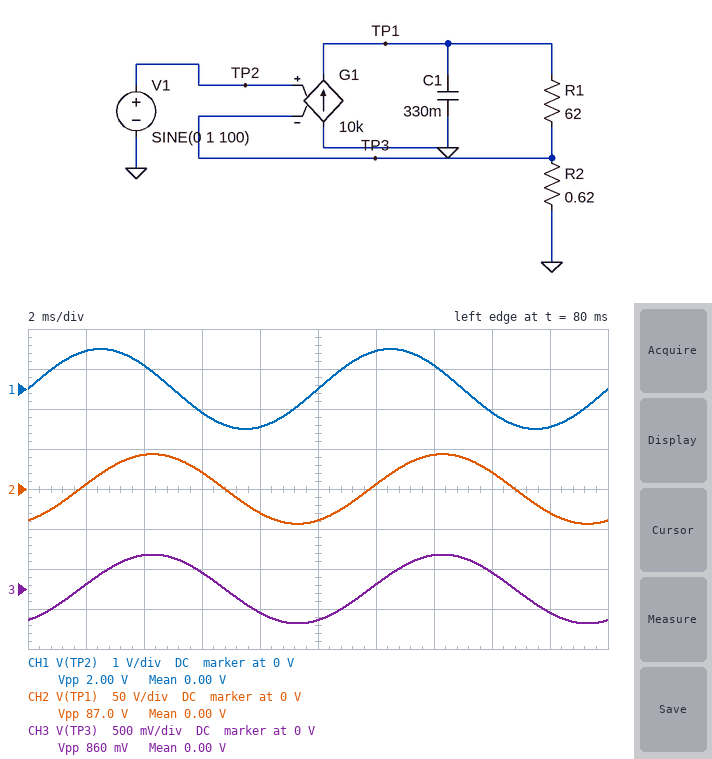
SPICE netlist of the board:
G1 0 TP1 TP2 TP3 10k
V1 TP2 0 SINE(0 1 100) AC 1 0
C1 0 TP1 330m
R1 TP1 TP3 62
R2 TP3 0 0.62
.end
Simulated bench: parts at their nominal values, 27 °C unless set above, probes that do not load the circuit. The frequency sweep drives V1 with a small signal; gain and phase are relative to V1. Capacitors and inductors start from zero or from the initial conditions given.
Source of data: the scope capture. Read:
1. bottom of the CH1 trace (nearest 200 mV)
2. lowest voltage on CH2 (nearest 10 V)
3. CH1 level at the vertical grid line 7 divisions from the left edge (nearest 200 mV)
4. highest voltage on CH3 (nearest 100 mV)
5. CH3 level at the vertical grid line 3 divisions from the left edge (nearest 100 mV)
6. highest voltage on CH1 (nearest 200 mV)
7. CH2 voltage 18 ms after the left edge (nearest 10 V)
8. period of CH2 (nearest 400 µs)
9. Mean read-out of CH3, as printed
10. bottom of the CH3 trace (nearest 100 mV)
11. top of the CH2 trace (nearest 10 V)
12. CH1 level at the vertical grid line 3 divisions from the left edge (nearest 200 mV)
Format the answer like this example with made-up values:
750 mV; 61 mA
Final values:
-1.0 V; -40 V; 600 mV; 400 mV; 200 mV; 1.0 V; -30 V; 10.0 ms; 0.00 V; -400 mV; 40 V; -600 mV
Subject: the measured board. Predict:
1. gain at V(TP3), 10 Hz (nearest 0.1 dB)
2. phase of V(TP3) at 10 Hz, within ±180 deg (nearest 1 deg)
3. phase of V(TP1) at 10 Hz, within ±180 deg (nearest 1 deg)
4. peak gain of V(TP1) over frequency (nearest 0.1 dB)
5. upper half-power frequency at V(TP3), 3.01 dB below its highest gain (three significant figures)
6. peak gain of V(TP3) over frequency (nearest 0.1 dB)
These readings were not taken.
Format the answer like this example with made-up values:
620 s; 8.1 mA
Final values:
-0.2 dB; -12 deg; -12 deg; 40.1 dB; 47.8 Hz; 0 dB
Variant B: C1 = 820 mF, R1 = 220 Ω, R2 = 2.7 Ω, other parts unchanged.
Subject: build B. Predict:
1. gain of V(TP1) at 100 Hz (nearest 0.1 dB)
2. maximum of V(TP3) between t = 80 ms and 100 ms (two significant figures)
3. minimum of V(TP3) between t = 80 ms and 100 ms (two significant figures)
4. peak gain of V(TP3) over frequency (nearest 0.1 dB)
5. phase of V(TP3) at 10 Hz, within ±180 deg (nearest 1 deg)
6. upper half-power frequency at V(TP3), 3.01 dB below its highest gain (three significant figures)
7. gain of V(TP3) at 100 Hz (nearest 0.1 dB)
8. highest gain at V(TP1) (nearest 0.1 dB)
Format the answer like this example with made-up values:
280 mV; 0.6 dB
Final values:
25.5 dB; 230 mV; -230 mV; 0 dB; -23 deg; 23.5 Hz; -12.8 dB; 38.3 dB
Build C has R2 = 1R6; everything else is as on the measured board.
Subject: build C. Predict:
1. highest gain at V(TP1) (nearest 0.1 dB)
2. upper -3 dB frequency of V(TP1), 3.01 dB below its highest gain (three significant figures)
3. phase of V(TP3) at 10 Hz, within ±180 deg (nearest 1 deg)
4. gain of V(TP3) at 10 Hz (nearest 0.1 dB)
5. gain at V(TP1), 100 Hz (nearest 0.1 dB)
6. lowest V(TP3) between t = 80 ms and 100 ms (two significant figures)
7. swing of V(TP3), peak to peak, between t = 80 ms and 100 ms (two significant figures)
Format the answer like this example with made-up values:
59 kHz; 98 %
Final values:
32.0 dB; 121 Hz; -5 deg; 0 dB; 29.7 dB; -770 mV; 1.5 V
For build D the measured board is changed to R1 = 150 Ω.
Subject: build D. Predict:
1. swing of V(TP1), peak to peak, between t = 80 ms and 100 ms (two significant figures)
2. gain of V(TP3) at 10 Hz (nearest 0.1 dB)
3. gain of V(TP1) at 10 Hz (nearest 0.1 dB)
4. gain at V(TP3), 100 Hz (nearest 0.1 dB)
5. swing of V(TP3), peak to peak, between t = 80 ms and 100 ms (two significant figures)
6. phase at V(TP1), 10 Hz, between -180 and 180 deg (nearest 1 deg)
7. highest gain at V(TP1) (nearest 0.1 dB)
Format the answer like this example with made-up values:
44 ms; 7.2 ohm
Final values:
95 V; -1.0 dB; 46.7 dB; -14.2 dB; 390 mV; -27 deg; 47.7 dB
